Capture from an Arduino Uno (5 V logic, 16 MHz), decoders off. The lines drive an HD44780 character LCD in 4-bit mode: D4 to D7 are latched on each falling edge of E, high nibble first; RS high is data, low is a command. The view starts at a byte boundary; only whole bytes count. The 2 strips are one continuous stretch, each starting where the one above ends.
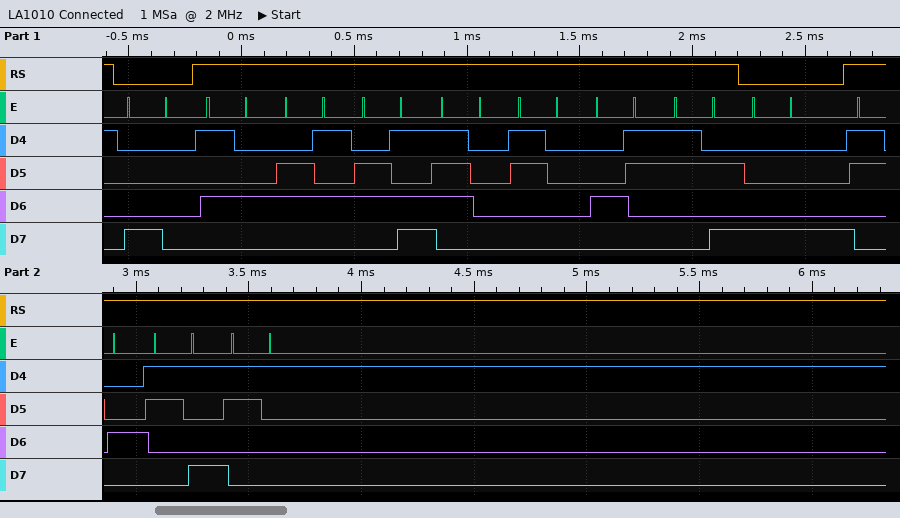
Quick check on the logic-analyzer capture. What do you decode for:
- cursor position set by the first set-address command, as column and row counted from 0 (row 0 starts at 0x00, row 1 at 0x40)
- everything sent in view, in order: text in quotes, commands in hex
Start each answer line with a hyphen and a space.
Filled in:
- column 0, row 0
- 0x80 "Temp0C:" 0x88 "491"
